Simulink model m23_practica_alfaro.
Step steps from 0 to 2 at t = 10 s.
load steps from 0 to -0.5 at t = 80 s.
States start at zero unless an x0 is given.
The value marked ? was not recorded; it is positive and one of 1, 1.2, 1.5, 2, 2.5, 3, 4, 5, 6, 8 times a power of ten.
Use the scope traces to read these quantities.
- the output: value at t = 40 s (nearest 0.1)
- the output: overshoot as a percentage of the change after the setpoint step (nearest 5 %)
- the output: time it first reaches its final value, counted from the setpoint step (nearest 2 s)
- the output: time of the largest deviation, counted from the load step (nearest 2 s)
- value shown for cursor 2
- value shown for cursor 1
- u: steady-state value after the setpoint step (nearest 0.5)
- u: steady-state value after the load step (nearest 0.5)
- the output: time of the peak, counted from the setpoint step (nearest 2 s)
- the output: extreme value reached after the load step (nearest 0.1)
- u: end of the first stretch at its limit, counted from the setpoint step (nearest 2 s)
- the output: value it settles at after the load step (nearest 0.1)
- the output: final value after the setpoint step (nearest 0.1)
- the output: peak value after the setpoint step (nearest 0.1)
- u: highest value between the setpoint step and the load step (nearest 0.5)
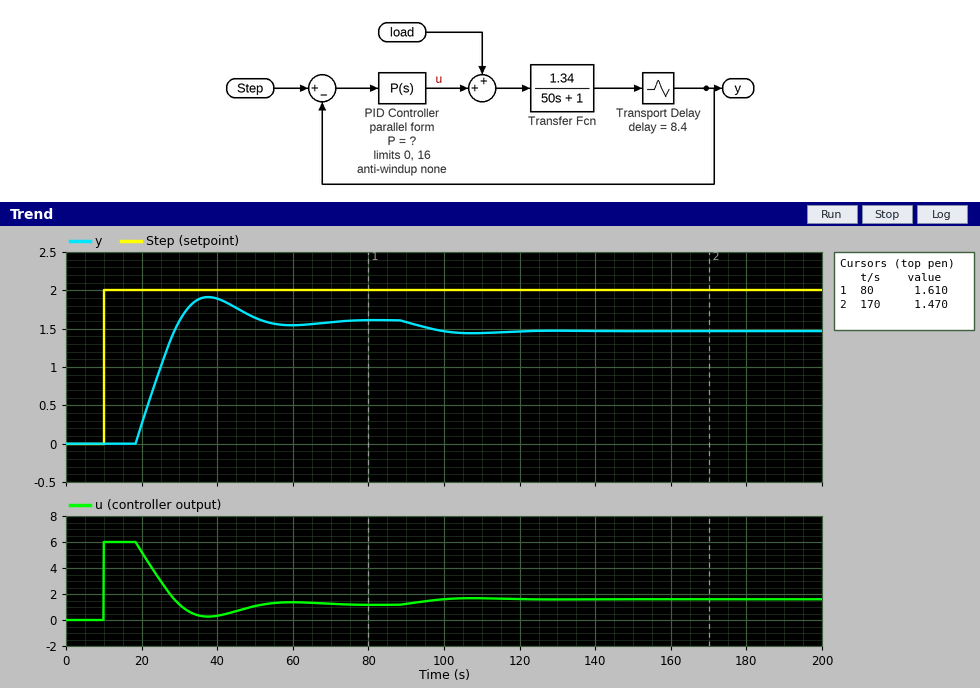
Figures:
1.9
20 %
20 s
28 s
1.470
1.610
1.0
1.5
28 s
1.4
8 s
1.5
1.6
1.9
6.0
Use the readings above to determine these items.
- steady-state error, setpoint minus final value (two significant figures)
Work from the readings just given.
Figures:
0.40
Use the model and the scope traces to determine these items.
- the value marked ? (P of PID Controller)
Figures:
3
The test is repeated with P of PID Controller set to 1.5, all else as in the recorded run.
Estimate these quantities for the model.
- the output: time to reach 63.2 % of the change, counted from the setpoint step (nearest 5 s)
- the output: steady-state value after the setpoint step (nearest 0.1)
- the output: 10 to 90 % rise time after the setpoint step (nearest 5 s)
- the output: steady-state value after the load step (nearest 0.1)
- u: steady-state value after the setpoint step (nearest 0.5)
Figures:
20 s
1.3
20 s
1.1
1.0
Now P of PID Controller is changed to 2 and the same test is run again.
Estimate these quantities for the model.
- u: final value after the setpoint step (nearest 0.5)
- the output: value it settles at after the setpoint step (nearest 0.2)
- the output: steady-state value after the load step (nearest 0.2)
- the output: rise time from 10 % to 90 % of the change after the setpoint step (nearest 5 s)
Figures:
1.0
1.4
1.2
15 s
